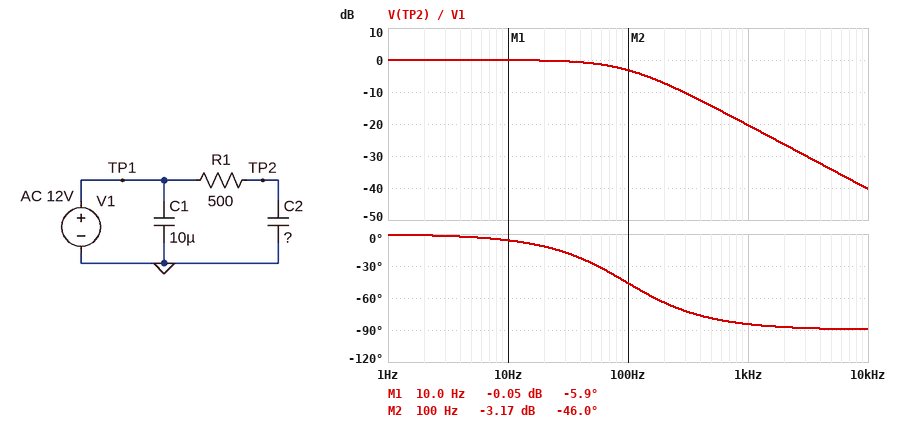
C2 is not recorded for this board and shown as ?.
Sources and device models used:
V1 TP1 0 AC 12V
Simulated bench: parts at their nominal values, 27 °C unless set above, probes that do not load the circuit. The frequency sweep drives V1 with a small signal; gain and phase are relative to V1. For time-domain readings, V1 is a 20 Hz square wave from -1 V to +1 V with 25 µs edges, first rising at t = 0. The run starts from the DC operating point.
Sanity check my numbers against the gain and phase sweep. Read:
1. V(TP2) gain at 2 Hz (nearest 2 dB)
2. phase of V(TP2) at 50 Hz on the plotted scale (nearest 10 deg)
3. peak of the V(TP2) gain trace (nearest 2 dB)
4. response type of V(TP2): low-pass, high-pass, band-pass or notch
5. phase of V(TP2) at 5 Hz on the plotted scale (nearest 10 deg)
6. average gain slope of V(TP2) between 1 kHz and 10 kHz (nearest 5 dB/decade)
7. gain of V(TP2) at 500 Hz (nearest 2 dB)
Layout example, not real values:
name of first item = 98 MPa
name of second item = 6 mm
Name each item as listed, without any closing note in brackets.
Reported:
V(TP2) gain at 2 Hz = 0 dB
phase of V(TP2) at 50 Hz on the plotted scale = -30 deg
peak of the V(TP2) gain trace = 0 dB
response type of V(TP2): low-pass, high-pass, band-pass or notch = low-pass
phase of V(TP2) at 5 Hz on the plotted scale = 0 deg
average gain slope of V(TP2) between 1 kHz and 10 kHz = -20 dB/decade
gain of V(TP2) at 500 Hz = -14 dB
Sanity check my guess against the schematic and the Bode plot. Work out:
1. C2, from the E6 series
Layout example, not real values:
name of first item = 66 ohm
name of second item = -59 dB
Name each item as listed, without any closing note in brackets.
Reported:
C2, from the E6 series = 3.3 µF
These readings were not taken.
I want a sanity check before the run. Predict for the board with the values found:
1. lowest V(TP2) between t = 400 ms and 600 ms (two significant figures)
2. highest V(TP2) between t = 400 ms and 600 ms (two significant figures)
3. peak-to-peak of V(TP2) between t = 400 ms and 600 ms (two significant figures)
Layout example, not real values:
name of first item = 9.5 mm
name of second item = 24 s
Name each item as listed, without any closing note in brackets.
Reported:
lowest V(TP2) between t = 400 ms and 600 ms = -1.0 V
highest V(TP2) between t = 400 ms and 600 ms = 1.0 V
peak-to-peak of V(TP2) between t = 400 ms and 600 ms = 2.0 V
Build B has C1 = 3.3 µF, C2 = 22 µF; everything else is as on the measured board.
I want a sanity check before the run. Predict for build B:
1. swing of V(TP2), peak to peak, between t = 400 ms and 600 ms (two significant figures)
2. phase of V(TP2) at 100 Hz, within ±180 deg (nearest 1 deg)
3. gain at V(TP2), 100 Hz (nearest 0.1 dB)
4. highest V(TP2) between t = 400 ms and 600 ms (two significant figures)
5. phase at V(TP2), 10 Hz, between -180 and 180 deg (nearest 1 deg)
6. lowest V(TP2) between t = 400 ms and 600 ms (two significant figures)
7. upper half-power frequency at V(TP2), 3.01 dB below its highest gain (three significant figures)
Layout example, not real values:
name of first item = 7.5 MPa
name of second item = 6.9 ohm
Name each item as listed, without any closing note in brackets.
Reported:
swing of V(TP2), peak to peak, between t = 400 ms and 600 ms = 1.6 V
phase of V(TP2) at 100 Hz, within ±180 deg = -82 deg
gain at V(TP2), 100 Hz = -16.9 dB
highest V(TP2) between t = 400 ms and 600 ms = 810 mV
phase at V(TP2), 10 Hz, between -180 and 180 deg = -35 deg
lowest V(TP2) between t = 400 ms and 600 ms = -810 mV
upper half-power frequency at V(TP2), 3.01 dB below its highest gain = 14.5 Hz
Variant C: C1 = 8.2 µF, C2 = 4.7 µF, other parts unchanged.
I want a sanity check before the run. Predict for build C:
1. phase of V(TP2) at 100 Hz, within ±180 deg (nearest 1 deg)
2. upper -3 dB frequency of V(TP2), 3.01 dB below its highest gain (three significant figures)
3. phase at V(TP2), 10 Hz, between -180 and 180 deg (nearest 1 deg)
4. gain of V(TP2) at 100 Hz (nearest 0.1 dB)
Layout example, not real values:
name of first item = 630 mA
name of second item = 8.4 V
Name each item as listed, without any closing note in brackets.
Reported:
phase of V(TP2) at 100 Hz, within ±180 deg = -56 deg
upper -3 dB frequency of V(TP2), 3.01 dB below its highest gain = 67.7 Hz
phase at V(TP2), 10 Hz, between -180 and 180 deg = -8 deg
gain of V(TP2) at 100 Hz = -5.0 dB
